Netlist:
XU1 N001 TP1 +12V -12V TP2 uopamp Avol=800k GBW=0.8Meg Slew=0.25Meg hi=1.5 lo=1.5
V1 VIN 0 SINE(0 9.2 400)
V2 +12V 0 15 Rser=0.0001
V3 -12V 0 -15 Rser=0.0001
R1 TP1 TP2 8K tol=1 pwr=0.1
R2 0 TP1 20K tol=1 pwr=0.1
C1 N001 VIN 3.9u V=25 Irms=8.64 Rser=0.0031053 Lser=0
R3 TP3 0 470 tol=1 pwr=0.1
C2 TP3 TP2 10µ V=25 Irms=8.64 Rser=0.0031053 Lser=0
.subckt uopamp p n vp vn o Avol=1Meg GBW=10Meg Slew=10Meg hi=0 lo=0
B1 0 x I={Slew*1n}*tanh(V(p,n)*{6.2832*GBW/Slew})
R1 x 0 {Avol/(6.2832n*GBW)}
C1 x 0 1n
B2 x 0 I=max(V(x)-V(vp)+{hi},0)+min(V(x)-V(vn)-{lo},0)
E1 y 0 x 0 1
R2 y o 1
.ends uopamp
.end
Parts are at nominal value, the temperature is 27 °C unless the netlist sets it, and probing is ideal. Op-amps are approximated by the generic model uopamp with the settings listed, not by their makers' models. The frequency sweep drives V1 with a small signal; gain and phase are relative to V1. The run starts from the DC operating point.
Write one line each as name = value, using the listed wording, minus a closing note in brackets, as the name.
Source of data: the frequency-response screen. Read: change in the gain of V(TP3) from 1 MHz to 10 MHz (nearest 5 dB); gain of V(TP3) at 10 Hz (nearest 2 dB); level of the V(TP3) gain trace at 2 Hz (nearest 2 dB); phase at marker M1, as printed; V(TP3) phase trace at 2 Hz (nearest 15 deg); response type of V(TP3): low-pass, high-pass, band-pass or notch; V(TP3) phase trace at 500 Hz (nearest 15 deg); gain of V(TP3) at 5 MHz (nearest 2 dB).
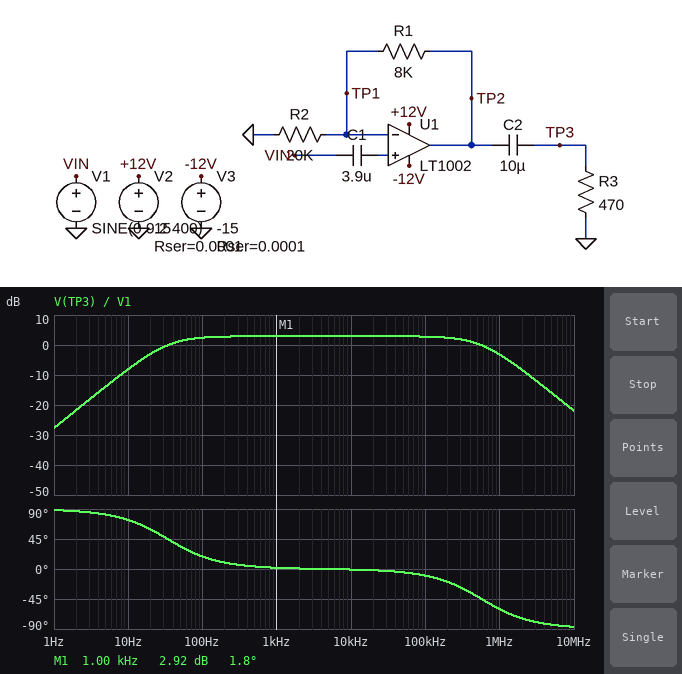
change in the gain of V(TP3) from 1 MHz to 10 MHz = -20 dB
gain of V(TP3) at 10 Hz = -8 dB
level of the V(TP3) gain trace at 2 Hz = -22 dB
phase at marker M1, as printed = 1.8 deg
V(TP3) phase trace at 2 Hz = 90 deg
response type of V(TP3): low-pass, high-pass, band-pass or notch = band-pass
V(TP3) phase trace at 500 Hz = 0 deg
gain of V(TP3) at 5 MHz = -16 dB
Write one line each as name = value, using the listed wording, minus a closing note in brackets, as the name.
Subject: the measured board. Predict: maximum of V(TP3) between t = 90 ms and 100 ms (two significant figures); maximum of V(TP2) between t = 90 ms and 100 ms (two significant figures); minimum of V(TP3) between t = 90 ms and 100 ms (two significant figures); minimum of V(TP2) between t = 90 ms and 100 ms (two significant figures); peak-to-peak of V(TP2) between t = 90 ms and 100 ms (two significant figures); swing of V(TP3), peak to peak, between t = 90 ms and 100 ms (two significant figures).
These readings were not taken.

maximum of V(TP3) between t = 90 ms and 100 ms = 13 V
maximum of V(TP2) between t = 90 ms and 100 ms = 13 V
minimum of V(TP3) between t = 90 ms and 100 ms = -13 V
minimum of V(TP2) between t = 90 ms and 100 ms = -13 V
peak-to-peak of V(TP2) between t = 90 ms and 100 ms = 26 V
swing of V(TP3), peak to peak, between t = 90 ms and 100 ms = 26 V
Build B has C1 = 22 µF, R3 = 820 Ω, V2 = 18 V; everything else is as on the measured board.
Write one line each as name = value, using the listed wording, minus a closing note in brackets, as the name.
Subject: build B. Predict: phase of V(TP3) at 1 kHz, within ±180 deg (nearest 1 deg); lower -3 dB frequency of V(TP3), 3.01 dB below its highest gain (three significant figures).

phase of V(TP3) at 1 kHz, within ±180 deg = 1 deg
lower -3 dB frequency of V(TP3), 3.01 dB below its highest gain = 19.4 Hz
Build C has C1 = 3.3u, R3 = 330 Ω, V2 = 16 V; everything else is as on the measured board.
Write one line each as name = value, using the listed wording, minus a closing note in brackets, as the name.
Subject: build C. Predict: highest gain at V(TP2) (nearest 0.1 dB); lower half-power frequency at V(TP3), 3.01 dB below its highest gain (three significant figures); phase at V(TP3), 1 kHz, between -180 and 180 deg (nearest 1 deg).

highest gain at V(TP2) = 2.9 dB
lower half-power frequency at V(TP3), 3.01 dB below its highest gain = 48.2 Hz
phase at V(TP3), 1 kHz, between -180 and 180 deg = 3 deg
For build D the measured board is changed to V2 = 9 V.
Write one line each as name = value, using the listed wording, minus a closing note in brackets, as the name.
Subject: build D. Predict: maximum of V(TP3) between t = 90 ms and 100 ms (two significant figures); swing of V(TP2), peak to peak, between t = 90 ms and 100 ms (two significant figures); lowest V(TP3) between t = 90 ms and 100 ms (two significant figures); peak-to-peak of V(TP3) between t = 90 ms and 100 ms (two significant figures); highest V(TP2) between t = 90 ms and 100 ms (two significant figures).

maximum of V(TP3) between t = 90 ms and 100 ms = 9.2 V
swing of V(TP2), peak to peak, between t = 90 ms and 100 ms = 20 V
lowest V(TP3) between t = 90 ms and 100 ms = -12 V
peak-to-peak of V(TP3) between t = 90 ms and 100 ms = 21 V
highest V(TP2) between t = 90 ms and 100 ms = 7.5 V
